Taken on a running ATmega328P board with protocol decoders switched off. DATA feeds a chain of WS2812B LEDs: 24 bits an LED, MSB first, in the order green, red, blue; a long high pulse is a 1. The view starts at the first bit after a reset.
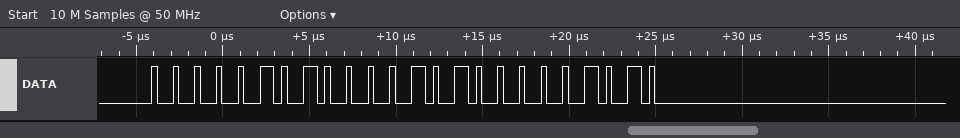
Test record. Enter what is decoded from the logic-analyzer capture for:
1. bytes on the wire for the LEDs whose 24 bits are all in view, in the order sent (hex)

05 0A 0A
